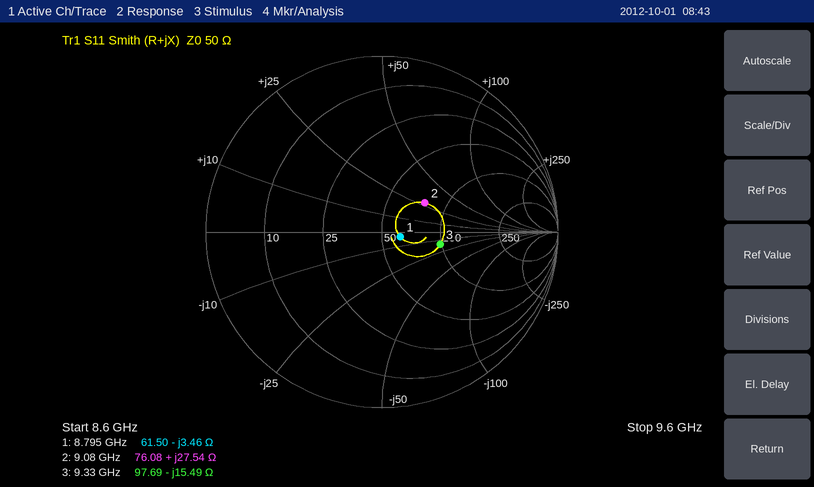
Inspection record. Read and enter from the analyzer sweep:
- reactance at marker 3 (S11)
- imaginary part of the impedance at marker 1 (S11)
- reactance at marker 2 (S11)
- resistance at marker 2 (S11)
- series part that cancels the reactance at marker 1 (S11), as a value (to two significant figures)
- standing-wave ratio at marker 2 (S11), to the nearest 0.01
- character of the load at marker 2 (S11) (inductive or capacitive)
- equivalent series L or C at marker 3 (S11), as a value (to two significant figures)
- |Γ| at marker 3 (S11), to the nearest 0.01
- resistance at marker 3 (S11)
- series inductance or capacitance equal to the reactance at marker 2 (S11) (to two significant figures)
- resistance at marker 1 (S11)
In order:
-15.49 Ω
-3.46 Ω
+27.54 Ω
76.08 Ω
63 pH
1.83
inductive
1.1 pF
0.34
97.69 Ω
480 pH
61.50 Ω
